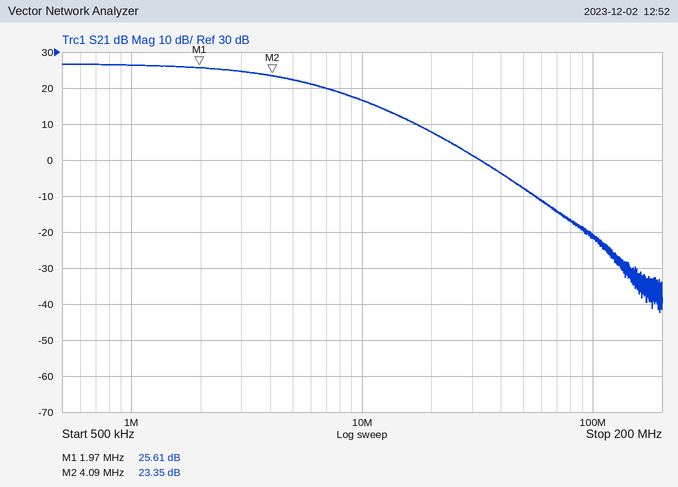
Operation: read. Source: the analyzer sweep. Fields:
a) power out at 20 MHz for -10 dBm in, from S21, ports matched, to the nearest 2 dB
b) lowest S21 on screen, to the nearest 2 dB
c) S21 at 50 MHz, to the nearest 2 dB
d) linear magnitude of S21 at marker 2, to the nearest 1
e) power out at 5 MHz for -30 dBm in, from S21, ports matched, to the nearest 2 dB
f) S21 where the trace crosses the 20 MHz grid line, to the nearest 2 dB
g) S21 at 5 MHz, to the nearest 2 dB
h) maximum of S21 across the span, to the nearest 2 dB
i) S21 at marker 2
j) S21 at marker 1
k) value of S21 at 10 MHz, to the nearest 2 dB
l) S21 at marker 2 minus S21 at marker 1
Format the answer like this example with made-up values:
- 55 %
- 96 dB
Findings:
- -2 dBm
- -42 dB
- -8 dB
- 15
- -8 dBm
- 8 dB
- 22 dB
- 26 dB
- 23.35 dB
- 25.61 dB
- 16 dB
- -2.26 dB
